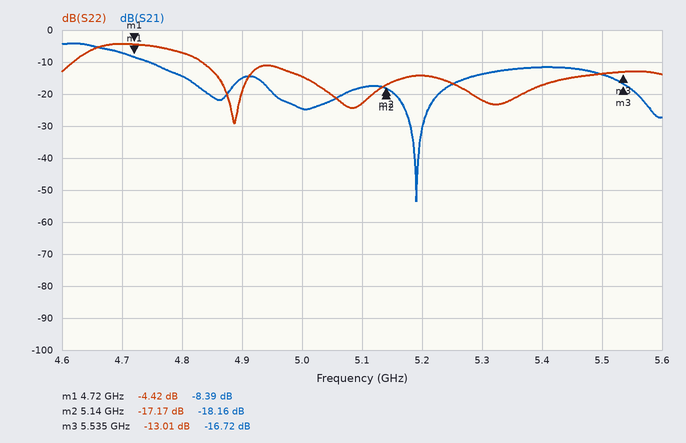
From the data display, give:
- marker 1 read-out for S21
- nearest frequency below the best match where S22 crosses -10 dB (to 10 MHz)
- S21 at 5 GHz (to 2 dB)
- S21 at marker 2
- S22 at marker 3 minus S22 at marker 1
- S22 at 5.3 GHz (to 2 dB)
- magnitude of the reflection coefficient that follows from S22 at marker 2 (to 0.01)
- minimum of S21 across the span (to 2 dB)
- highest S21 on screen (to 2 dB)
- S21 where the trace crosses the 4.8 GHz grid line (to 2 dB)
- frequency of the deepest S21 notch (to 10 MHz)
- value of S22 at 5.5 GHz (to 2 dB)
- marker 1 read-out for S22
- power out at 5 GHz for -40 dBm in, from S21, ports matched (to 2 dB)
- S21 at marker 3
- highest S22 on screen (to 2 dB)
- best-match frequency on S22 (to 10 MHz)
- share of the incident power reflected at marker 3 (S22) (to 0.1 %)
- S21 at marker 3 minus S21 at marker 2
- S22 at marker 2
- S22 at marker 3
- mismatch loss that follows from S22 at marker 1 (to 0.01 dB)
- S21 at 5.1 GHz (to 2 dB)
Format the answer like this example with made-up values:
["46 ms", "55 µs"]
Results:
["-8.39 dB", "4.83 GHz", "-24 dB", "-18.16 dB", "-8.59 dB", "-22 dB", "0.14", "-54 dB", "-4 dB", "-14 dB", "5.19 GHz", "-14 dB", "-4.42 dB", "-64 dBm", "-16.72 dB", "-4 dB", "4.89 GHz", "5.0 %", "1.44 dB", "-17.17 dB", "-13.01 dB", "1.95 dB", "-18 dB"]
